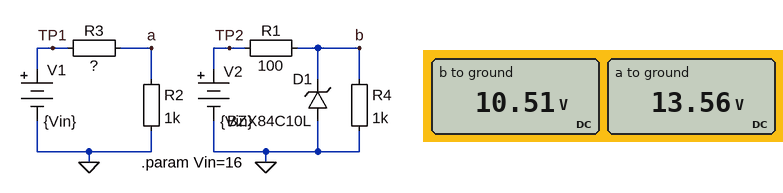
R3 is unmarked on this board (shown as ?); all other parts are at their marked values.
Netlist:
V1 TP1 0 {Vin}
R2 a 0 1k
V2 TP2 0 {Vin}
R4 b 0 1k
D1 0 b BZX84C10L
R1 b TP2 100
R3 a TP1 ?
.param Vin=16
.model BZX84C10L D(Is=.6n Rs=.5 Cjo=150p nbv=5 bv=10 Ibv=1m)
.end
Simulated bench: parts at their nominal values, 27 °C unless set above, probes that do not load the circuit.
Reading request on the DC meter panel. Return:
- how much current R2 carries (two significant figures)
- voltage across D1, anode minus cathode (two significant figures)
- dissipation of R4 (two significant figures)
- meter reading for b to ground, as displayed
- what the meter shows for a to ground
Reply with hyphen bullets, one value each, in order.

- 14 mA
- -11 V
- 110 mW
- 10.51 V
- 13.56 V
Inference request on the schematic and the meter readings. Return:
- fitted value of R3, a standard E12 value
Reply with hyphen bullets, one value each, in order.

- 180 Ω
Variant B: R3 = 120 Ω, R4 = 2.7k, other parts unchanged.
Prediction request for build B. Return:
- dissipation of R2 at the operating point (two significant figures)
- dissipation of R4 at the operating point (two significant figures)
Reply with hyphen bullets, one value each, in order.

- 200 mW
- 41 mW
